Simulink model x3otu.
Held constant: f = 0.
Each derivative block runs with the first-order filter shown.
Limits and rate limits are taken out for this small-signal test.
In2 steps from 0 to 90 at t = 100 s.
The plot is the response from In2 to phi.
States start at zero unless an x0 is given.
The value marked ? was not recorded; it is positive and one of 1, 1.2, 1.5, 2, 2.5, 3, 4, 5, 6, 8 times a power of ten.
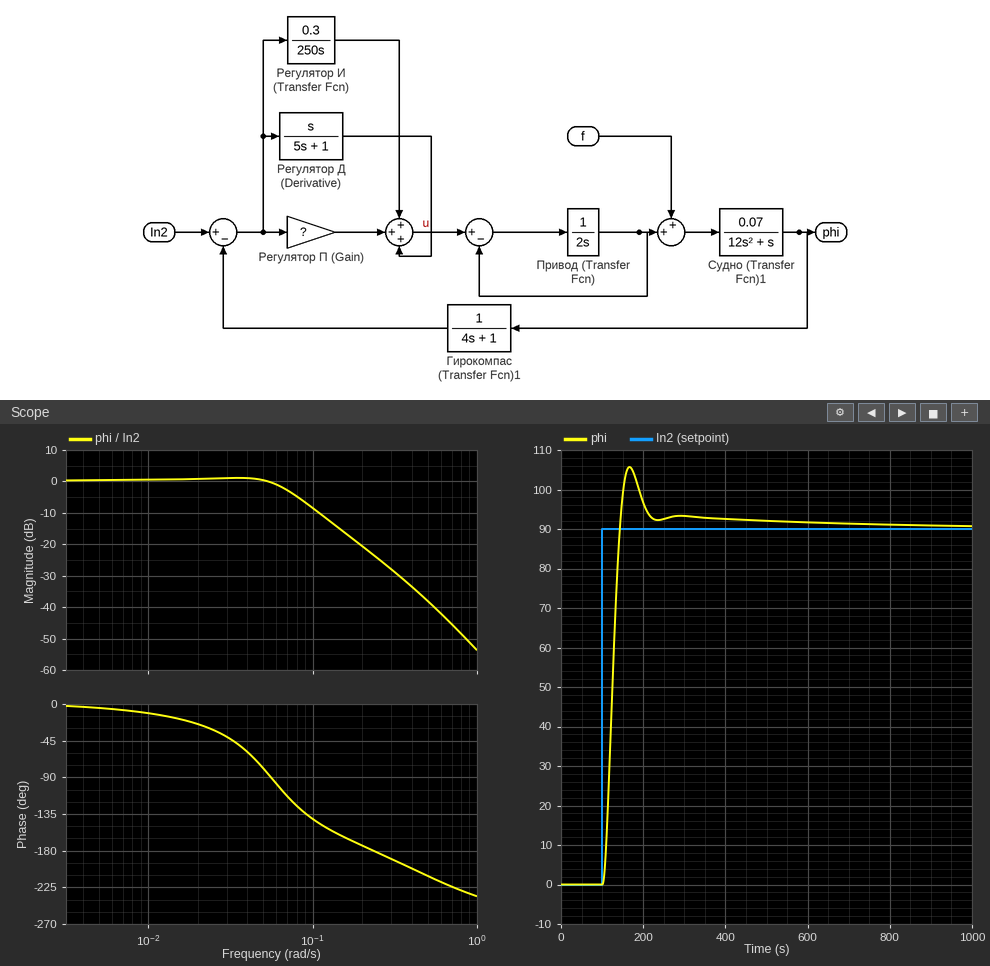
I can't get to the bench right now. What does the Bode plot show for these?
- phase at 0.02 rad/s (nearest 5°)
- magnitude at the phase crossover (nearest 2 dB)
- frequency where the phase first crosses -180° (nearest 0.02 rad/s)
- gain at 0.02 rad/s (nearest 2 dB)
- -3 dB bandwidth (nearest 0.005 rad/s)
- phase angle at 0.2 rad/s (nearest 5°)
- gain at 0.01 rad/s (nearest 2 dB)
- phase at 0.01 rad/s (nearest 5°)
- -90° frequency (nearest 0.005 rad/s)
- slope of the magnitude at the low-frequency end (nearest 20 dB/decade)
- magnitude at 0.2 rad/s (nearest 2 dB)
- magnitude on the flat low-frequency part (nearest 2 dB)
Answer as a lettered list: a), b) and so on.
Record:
a) -25°
b) -24 dB
c) 0.24 rad/s
d) 0 dB
e) 0.070 rad/s
f) -175°
g) 0 dB
h) -10°
i) 0.055 rad/s
j) 0 dB/decade
k) -20 dB
l) 0 dB
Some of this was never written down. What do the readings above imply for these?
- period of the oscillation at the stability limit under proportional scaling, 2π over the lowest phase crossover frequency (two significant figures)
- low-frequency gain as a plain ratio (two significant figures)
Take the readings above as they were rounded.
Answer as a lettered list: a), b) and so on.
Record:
a) 26 s
b) 1.0
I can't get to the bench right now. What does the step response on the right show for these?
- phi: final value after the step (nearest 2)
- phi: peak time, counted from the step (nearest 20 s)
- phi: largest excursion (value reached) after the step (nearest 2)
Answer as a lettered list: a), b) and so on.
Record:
a) 90
b) 60 s
c) 106
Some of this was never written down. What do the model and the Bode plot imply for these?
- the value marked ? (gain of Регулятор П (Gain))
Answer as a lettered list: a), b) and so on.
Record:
a) 0.6
